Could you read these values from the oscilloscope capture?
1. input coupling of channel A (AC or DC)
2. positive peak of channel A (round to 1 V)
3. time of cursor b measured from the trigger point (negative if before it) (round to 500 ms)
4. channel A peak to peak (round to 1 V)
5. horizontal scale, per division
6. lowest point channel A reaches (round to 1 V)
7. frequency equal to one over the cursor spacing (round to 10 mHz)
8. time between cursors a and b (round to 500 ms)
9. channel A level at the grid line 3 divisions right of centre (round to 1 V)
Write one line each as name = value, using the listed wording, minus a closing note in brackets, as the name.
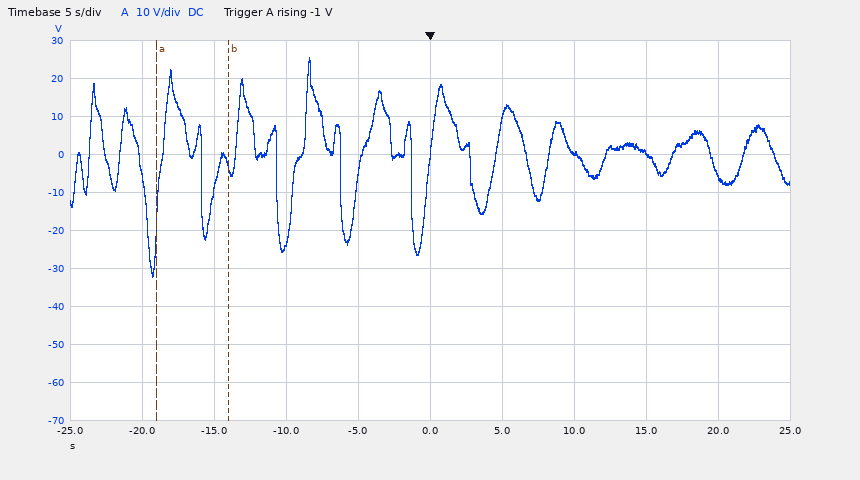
input coupling of channel A = DC
positive peak of channel A = 26 V
time of cursor b measured from the trigger point (negative if before it) = -14.0 s
channel A peak to peak = 58 V
horizontal scale, per division = 5 s
lowest point channel A reaches = -32 V
frequency equal to one over the cursor spacing = 200 mHz
time between cursors a and b = 5.0 s
channel A level at the grid line 3 divisions right of centre = 0 V
